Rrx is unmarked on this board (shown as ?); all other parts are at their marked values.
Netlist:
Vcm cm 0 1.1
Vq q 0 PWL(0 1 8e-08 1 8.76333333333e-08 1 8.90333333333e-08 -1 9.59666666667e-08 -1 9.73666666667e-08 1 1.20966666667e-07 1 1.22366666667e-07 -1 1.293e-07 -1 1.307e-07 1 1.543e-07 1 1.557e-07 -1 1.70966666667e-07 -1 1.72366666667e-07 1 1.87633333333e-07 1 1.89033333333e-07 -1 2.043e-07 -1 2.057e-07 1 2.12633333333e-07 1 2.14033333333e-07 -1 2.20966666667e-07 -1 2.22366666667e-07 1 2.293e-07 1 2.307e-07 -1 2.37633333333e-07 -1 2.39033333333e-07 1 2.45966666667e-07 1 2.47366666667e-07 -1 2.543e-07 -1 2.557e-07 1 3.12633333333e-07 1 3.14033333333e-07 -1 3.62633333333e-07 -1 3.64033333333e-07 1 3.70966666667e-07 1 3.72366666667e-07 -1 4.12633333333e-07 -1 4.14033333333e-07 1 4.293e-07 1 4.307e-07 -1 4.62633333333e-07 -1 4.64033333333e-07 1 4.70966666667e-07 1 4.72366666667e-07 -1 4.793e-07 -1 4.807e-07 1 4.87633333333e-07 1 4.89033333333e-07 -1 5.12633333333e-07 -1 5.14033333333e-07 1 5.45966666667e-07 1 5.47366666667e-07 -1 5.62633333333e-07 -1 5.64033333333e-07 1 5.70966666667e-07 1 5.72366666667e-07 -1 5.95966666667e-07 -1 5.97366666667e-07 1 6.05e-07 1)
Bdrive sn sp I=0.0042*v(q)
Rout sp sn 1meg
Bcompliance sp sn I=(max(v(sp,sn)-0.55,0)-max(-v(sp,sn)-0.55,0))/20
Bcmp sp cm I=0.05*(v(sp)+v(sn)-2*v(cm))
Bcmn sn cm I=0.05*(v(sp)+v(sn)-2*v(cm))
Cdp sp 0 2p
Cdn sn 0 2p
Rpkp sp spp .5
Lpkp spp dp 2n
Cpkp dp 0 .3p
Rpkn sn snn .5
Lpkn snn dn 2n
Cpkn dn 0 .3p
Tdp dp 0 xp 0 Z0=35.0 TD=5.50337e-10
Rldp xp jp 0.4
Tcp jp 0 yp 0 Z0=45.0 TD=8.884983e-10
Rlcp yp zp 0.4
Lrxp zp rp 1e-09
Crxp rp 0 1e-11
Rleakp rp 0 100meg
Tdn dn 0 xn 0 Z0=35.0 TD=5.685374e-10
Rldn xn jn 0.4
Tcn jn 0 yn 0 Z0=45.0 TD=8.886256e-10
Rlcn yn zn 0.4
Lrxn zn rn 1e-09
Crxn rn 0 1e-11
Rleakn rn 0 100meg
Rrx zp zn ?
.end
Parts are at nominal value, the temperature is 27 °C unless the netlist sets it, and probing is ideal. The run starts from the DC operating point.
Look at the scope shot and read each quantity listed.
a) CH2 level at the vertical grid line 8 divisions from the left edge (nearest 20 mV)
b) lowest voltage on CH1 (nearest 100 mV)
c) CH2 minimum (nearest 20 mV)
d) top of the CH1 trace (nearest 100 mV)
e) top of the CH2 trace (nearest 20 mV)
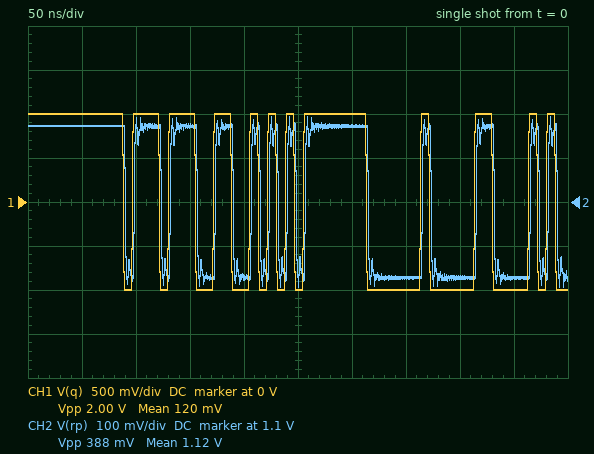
920 mV
-1.0 V
900 mV
1.0 V
1.30 V
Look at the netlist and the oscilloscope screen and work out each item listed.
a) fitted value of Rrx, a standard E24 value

82 Ω
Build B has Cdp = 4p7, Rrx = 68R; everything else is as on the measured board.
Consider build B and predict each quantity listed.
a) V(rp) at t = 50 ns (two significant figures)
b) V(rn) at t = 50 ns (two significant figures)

1.2 V
960 mV
